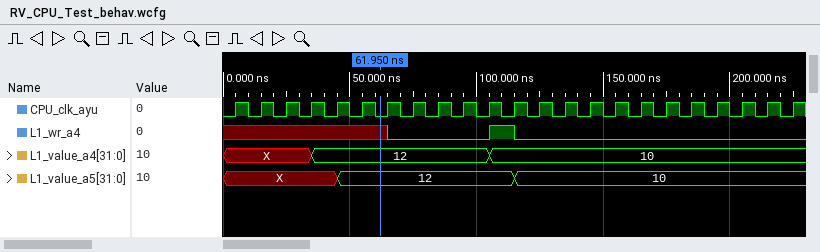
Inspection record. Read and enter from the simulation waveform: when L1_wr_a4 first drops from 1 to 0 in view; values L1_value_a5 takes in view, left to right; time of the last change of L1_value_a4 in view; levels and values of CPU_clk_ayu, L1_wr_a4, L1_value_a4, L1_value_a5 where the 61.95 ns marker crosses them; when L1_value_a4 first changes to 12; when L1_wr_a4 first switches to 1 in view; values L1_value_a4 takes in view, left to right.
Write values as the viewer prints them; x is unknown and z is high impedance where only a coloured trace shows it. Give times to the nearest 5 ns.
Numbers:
115 ns
X, 12, 10
105 ns
CPU_clk_ayu=0, L1_wr_a4=x, L1_value_a4=12, L1_value_a5=12
35 ns
105 ns
X, 12, 10
